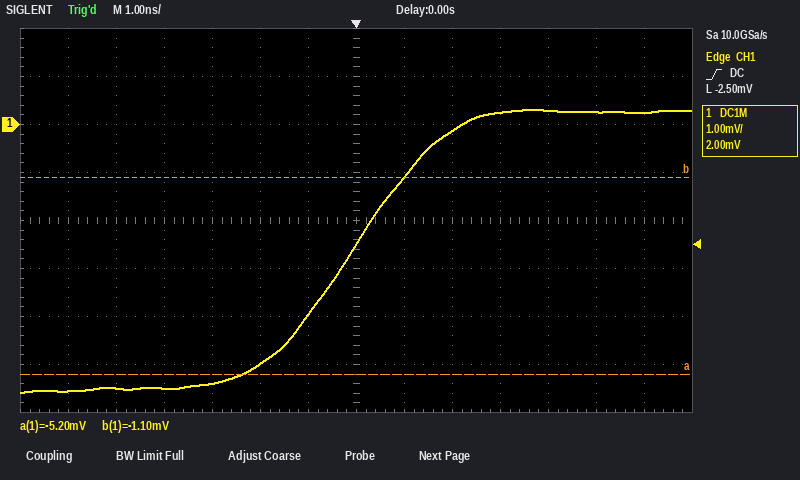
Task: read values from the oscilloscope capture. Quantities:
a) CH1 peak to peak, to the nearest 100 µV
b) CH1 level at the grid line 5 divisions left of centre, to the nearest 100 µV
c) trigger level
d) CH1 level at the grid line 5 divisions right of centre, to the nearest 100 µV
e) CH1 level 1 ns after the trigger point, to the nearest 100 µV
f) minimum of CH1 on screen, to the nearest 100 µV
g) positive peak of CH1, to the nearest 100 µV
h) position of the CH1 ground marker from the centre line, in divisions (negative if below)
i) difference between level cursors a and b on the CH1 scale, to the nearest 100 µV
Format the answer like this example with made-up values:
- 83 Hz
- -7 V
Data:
- 5.9 mV
- -5.5 mV
- -2.50 mV
- 300 µV
- -1.1 mV
- -5.6 mV
- 300 µV
- +2.0 div
- 4.1 mV
